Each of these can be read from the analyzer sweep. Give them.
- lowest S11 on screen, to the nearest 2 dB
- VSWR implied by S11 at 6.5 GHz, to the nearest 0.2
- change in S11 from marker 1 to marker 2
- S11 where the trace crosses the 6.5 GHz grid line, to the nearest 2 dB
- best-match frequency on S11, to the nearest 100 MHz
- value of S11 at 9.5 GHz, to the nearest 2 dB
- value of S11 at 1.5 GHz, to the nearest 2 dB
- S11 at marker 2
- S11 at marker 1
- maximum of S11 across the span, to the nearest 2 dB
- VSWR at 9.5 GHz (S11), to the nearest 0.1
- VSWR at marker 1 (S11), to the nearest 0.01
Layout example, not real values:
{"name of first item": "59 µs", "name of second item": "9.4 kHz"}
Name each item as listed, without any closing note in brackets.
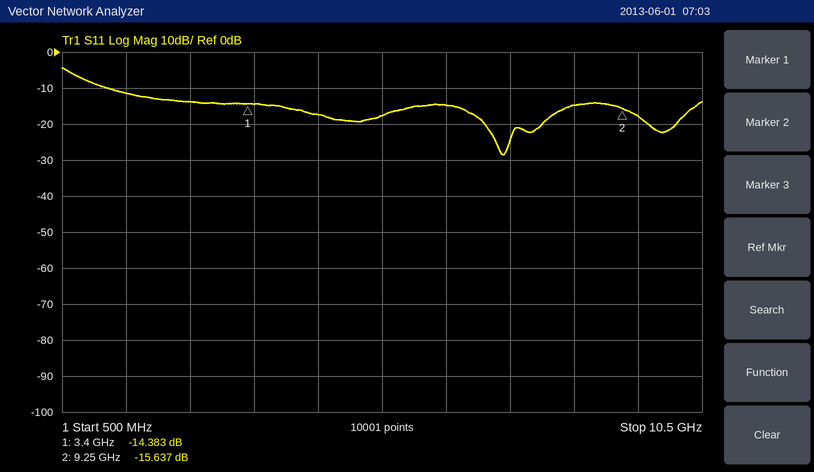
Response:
{"lowest S11 on screen, to the nearest 2 dB": "-28 dB", "VSWR implied by S11 at 6.5 GHz, to the nearest 0.2": "1.4", "change in S11 from marker 1 to marker 2": "-1.254 dB", "S11 where the trace crosses the 6.5 GHz grid line, to the nearest 2 dB": "-14 dB", "best-match frequency on S11, to the nearest 100 MHz": "7.4 GHz", "value of S11 at 9.5 GHz, to the nearest 2 dB": "-18 dB", "value of S11 at 1.5 GHz, to the nearest 2 dB": "-12 dB", "S11 at marker 2": "-15.637 dB", "S11 at marker 1": "-14.383 dB", "maximum of S11 across the span, to the nearest 2 dB": "-4 dB", "VSWR at 9.5 GHz (S11), to the nearest 0.1": "1.3", "VSWR at marker 1 (S11), to the nearest 0.01": "1.47"}
